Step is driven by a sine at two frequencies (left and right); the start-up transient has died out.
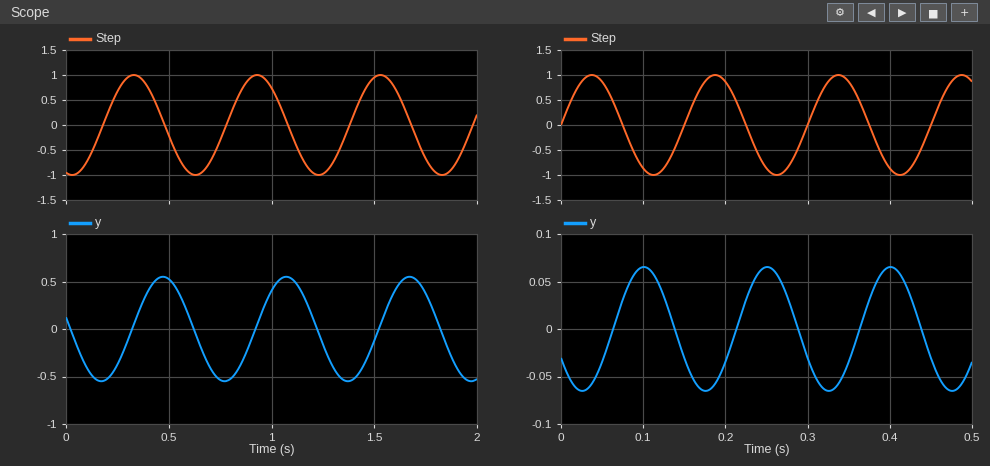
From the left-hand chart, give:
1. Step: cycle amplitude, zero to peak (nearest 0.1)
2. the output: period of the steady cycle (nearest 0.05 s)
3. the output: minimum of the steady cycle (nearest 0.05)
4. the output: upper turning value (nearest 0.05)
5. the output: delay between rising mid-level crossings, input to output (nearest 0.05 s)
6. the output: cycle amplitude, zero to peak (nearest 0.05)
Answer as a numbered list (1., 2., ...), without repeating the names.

1. 1.0
2. 0.60 s
3. -0.55
4. 0.55
5. 0.15 s
6. 0.55
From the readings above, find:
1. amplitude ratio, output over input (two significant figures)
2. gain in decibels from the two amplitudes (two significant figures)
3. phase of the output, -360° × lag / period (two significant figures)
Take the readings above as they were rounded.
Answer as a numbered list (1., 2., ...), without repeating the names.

1. 0.55
2. -5.2 dB
3. -90°
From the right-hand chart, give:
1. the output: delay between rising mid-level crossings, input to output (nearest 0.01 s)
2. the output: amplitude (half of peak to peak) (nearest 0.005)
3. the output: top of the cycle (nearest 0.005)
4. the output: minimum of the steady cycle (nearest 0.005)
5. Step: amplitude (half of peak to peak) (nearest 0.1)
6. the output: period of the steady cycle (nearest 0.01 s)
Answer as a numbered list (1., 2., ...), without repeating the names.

1. 0.06 s
2. 0.065
3. 0.065
4. -0.065
5. 1.0
6. 0.15 s
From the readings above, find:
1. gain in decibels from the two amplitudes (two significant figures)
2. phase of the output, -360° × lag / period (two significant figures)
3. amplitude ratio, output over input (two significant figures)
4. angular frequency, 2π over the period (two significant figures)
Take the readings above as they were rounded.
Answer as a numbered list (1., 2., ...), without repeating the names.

1. -24 dB
2. -140°
3. 0.065
4. 42 rad/s
